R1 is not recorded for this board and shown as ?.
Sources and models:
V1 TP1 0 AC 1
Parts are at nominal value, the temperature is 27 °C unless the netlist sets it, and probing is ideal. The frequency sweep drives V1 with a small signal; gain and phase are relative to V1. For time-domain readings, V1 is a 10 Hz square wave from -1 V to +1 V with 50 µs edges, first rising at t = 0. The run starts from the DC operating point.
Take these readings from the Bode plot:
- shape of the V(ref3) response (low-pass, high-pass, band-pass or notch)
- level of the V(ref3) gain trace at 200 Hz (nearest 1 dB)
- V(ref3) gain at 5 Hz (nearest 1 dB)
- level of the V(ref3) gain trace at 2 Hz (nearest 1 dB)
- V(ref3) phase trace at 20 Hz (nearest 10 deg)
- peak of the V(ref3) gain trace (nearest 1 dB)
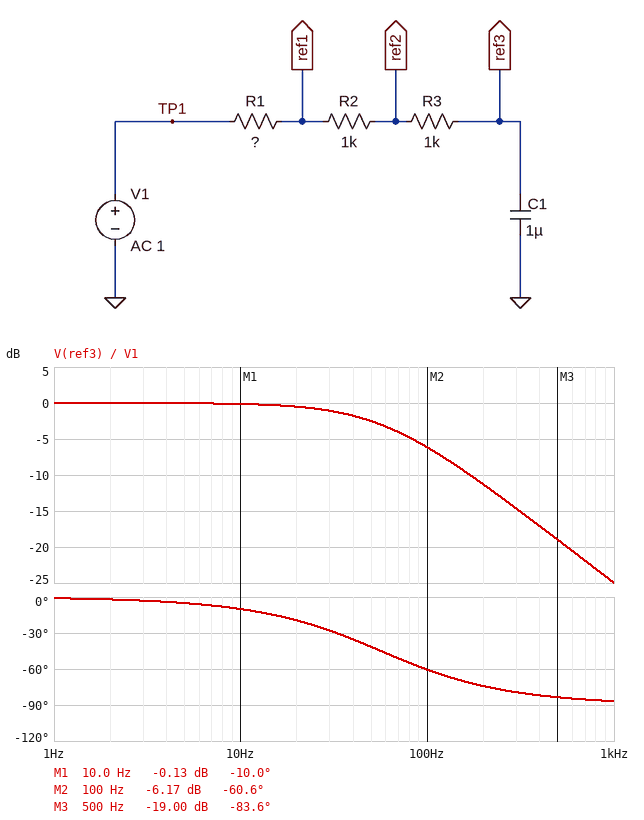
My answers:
low-pass
-11 dB
0 dB
0 dB
-20 deg
0 dB
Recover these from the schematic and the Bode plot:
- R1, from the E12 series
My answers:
820 Ω
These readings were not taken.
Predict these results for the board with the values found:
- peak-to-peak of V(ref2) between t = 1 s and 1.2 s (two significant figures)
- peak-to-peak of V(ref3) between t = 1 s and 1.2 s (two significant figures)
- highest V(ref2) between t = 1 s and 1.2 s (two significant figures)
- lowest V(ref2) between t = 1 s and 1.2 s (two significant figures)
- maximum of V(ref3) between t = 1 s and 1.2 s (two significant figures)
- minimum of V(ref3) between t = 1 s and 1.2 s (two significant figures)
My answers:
2.0 V
2.0 V
1.0 V
-1.0 V
1.0 V
-1.0 V
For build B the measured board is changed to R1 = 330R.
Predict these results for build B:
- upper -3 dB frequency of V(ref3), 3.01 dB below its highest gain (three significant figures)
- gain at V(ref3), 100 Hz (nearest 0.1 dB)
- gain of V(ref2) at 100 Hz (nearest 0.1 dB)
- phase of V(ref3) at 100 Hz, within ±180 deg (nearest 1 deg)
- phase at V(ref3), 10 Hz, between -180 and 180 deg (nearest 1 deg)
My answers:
68.3 Hz
-5.0 dB
-3.5 dB
-56 deg
-8 deg
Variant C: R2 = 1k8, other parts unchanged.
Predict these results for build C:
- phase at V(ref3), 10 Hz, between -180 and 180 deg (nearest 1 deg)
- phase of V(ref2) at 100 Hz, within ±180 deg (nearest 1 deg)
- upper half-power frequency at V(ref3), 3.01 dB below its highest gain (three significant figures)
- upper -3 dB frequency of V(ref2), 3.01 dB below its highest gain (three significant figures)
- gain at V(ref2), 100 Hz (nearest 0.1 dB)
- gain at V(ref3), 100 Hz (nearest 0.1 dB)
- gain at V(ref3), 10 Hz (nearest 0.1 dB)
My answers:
-13 deg
-34 deg
44.0 Hz
47.8 Hz
-6.5 dB
-7.9 dB
-0.2 dB
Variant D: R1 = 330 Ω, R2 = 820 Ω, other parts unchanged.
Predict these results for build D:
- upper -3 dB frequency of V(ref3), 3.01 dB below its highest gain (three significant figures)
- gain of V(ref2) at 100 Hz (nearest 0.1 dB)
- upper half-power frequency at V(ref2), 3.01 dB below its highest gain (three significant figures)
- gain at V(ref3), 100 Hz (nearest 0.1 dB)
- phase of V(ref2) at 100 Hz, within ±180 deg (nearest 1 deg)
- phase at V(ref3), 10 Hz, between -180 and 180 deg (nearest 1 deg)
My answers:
74.0 Hz
-3.1 dB
98.3 Hz
-4.5 dB
-21 deg
-8 deg
